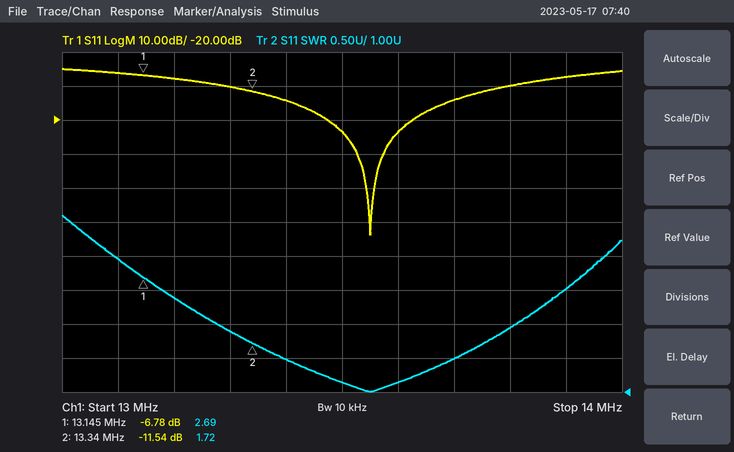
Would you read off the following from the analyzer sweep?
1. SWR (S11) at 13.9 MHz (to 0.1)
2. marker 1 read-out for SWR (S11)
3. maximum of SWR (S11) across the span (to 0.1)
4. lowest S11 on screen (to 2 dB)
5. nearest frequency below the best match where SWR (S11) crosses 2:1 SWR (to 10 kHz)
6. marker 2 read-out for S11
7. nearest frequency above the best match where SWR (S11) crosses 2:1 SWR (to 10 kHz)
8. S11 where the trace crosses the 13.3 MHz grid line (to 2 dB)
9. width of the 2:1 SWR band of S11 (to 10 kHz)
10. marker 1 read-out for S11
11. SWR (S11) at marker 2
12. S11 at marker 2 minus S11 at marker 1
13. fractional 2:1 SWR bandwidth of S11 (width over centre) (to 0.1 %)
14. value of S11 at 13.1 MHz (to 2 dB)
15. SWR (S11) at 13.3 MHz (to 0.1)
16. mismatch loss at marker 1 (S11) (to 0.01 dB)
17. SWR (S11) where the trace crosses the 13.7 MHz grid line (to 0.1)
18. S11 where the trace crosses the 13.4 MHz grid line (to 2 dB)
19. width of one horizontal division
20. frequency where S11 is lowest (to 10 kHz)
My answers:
2.5
2.69
3.6
-54 dB
13.28 MHz
-11.54 dB
13.81 MHz
-10 dB
530 kHz
-6.78 dB
1.72
-4.76 dB
3.9 %
-6 dB
1.9
1.02 dB
1.5
-14 dB
100 kHz
13.55 MHz
